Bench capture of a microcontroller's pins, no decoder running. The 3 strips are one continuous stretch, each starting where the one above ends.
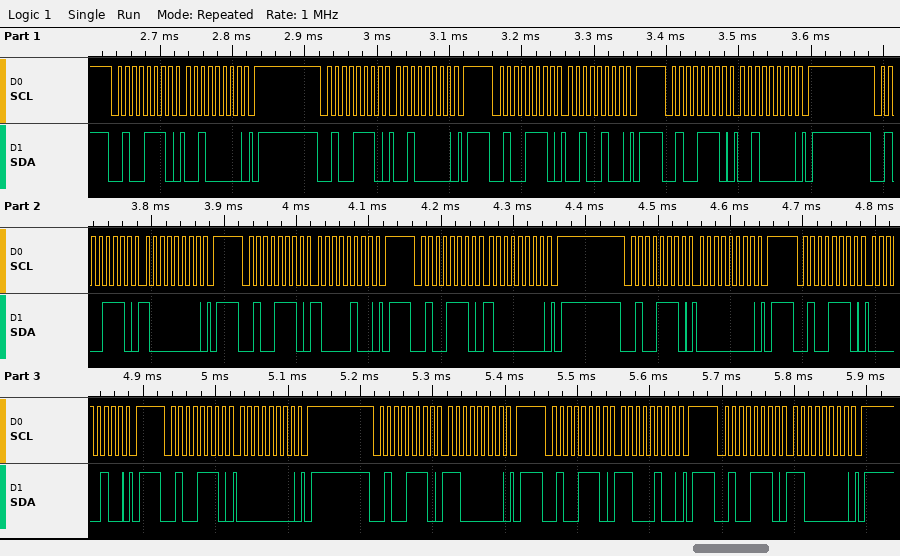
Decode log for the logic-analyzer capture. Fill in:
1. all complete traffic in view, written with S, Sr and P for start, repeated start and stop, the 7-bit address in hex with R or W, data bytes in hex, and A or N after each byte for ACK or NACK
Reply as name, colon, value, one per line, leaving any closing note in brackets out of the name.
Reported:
all complete traffic in view, written with S, Sr and P for start, repeated start and stop, the 7-bit address in hex with R or W, data bytes in hex, and A or N after each byte for ACK or NACK: S 27W A 20 A P S 27W A 20 A P S 27W A 24 A P S 27W A 20 A P S 27W A 80 A P S 27W A 84 A P S 27W A 80 A P S 27W A 00 A P S 27W A 04 A P S 27W A 00 A P S 27W A C0 A P S 27W A C4 A P S 27W A C0 A P
